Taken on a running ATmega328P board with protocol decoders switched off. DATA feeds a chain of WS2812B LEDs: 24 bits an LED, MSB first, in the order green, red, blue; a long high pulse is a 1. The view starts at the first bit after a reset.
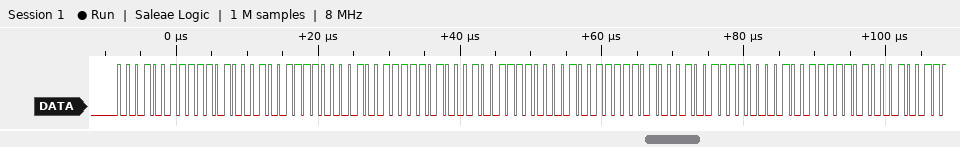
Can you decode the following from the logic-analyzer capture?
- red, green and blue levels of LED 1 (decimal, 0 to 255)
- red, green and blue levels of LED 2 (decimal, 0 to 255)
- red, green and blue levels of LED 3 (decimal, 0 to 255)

232, 19, 158
232, 19, 158
232, 19, 158
